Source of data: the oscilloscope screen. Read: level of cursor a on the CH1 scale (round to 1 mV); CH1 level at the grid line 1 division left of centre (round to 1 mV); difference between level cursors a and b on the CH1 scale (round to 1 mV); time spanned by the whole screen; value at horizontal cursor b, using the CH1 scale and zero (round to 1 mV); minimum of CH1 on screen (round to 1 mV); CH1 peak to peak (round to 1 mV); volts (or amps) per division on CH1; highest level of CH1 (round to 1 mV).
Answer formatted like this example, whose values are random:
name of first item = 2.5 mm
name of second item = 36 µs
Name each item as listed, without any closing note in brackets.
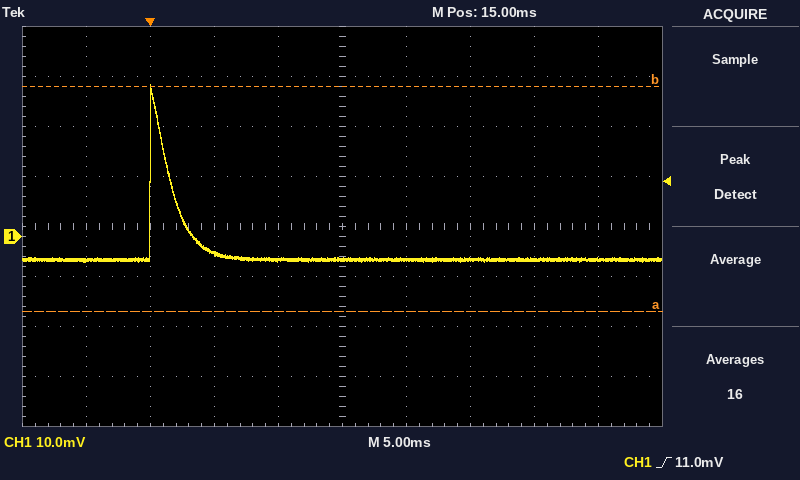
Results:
level of cursor a on the CH1 scale = -15 mV
CH1 level at the grid line 1 division left of centre = -5 mV
difference between level cursors a and b on the CH1 scale = 45 mV
time spanned by the whole screen = 50 ms
value at horizontal cursor b, using the CH1 scale and zero = 30 mV
minimum of CH1 on screen = -5 mV
CH1 peak to peak = 35 mV
volts (or amps) per division on CH1 = 10 mV
highest level of CH1 = 30 mV
